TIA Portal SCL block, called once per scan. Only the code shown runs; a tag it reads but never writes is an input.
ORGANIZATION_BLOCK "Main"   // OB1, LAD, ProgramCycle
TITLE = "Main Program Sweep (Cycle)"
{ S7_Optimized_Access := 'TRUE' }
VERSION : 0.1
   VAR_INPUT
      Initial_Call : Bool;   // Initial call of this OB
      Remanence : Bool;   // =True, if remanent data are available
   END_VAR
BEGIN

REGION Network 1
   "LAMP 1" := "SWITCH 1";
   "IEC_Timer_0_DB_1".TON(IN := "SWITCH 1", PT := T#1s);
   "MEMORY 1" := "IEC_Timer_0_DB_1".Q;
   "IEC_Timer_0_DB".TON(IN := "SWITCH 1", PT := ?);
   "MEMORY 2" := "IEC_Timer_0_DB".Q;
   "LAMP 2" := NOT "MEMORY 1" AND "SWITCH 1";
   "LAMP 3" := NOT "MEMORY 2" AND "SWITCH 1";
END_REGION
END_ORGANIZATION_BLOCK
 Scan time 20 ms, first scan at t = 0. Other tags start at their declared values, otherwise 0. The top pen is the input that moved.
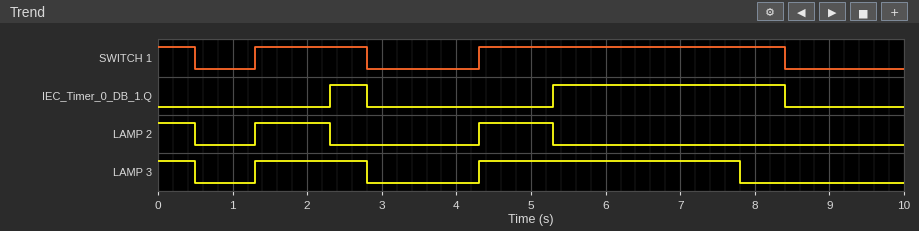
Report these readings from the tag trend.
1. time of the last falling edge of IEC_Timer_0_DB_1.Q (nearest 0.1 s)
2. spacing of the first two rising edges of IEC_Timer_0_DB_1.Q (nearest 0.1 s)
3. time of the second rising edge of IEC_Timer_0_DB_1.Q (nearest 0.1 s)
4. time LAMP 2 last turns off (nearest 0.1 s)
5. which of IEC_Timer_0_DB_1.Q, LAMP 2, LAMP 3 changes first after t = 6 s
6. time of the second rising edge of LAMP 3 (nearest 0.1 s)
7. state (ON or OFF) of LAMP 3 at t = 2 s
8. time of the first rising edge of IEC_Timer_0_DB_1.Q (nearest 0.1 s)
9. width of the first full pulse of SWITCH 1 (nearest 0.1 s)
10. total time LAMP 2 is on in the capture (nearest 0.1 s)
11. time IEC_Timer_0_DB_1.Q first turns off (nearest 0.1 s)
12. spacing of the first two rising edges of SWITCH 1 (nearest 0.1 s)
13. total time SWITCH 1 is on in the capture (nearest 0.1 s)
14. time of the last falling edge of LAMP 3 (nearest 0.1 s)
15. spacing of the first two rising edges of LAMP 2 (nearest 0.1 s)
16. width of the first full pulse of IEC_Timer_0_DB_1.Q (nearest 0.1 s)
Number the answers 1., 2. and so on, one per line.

1. 8.4 s
2. 3.0 s
3. 5.3 s
4. 5.3 s
5. LAMP 3
6. 4.3 s
7. ON
8. 2.3 s
9. 1.5 s
10. 2.5 s
11. 2.8 s
12. 3.0 s
13. 6.1 s
14. 7.8 s
15. 3.0 s
16. 0.5 s
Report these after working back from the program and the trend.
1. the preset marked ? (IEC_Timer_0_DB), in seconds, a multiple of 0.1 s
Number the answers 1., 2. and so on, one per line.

1. 3.5 s
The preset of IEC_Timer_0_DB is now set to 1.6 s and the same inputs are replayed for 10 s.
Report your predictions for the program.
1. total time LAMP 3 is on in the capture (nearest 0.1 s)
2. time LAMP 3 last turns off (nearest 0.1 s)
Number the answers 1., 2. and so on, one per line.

1. 3.6 s
2. 5.9 s
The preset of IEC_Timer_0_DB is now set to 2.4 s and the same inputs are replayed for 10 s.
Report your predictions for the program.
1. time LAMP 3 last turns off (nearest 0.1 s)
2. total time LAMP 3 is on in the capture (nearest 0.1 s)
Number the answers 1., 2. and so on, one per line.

1. 6.7 s
2. 4.4 s
